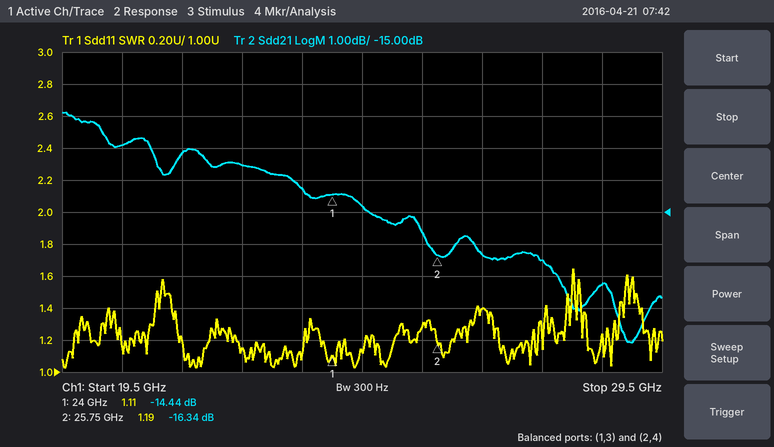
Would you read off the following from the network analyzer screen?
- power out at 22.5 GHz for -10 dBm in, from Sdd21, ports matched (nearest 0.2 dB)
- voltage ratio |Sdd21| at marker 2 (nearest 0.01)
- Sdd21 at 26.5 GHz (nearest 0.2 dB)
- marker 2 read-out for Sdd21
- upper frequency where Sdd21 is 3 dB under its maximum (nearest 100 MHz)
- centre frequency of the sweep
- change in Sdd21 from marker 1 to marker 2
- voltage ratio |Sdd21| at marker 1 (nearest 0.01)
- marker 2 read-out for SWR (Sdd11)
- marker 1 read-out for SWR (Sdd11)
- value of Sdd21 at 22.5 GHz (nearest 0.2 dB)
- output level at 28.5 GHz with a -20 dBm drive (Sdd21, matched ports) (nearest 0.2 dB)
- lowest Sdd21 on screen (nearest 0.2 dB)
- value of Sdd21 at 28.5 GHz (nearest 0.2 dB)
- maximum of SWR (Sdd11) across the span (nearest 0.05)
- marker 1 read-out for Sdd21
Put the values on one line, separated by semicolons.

-23.6 dBm; 0.15; -16.4 dB; -16.34 dB; 24.5 GHz; 24.5 GHz; -1.90 dB; 0.19; 1.19; 1.11; -13.6 dB; -37.2 dBm; -19.0 dB; -17.2 dB; 1.65; -14.44 dB
